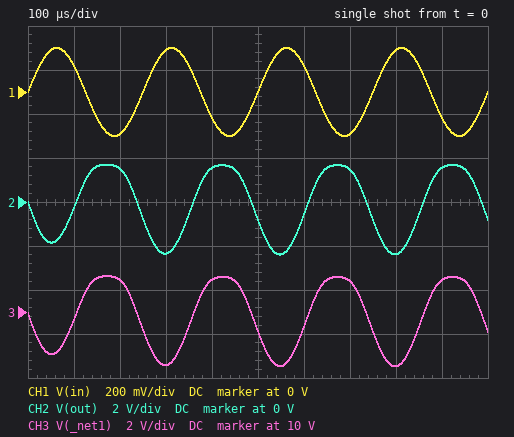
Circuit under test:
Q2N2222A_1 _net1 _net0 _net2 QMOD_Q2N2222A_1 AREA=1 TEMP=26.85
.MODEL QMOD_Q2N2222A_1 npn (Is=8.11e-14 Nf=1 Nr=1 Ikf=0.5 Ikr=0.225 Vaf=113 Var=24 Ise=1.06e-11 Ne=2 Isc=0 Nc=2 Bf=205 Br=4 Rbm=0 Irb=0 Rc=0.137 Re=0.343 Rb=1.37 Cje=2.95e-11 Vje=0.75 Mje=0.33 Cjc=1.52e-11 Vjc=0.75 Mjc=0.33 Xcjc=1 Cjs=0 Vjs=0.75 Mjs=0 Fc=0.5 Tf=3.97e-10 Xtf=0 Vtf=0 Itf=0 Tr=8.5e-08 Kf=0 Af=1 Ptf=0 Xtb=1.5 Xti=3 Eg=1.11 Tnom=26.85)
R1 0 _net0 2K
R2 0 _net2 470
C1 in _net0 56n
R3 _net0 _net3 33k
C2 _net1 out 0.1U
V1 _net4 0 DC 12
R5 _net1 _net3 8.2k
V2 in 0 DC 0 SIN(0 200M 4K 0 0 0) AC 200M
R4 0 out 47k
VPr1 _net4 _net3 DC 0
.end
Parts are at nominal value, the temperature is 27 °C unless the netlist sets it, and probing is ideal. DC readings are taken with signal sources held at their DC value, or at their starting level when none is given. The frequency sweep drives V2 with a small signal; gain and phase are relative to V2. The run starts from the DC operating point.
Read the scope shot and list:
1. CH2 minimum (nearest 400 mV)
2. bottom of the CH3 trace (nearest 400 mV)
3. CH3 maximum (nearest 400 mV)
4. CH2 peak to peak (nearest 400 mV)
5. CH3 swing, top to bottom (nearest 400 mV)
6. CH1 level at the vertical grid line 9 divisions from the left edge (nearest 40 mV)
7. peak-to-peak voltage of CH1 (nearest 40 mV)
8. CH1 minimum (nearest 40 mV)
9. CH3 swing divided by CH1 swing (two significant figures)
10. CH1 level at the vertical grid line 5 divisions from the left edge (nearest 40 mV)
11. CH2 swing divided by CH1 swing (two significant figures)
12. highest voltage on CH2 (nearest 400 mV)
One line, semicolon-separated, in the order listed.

-2.4 V; 7.6 V; 11.6 V; 4.0 V; 4.0 V; -120 mV; 400 mV; -200 mV; 10; 0 V; 10; 1.6 V
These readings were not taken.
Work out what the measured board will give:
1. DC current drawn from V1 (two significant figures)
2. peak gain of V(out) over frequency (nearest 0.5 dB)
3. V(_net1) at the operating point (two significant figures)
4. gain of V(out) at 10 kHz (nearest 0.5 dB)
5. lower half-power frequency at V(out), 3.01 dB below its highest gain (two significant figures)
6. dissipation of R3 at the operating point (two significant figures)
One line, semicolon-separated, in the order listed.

590 µA; 21.5 dB; 9.9 V; 21.5 dB; 1.5 kHz; 3.9 mW
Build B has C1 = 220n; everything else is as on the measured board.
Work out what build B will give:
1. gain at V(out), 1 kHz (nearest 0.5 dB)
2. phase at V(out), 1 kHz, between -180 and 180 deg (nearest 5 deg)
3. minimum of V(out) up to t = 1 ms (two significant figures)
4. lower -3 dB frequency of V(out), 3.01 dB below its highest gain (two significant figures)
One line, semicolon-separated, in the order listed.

21.0 dB; -155 deg; -2.5 V; 390 Hz
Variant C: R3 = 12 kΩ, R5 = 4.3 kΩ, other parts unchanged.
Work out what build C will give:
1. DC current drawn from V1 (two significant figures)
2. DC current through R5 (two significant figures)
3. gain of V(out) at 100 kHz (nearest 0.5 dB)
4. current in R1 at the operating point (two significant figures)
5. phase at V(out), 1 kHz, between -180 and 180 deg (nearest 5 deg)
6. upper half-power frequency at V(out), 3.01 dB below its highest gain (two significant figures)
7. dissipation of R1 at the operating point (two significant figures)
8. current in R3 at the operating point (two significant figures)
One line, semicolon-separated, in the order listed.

3.1 mA; 2.3 mA; 18.0 dB; 850 µA; -120 deg; 3.3 MHz; 1.4 mW; 860 µA
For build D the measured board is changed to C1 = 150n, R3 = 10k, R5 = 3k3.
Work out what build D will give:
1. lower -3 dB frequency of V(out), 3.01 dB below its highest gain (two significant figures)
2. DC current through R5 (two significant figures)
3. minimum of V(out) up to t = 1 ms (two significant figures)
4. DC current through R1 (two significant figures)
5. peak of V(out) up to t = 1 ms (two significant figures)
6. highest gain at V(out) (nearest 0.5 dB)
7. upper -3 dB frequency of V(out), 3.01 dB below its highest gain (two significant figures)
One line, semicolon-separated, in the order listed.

650 Hz; 2.8 mA; -1.0 V; 990 µA; 1.4 V; 16.0 dB; 4.3 MHz
